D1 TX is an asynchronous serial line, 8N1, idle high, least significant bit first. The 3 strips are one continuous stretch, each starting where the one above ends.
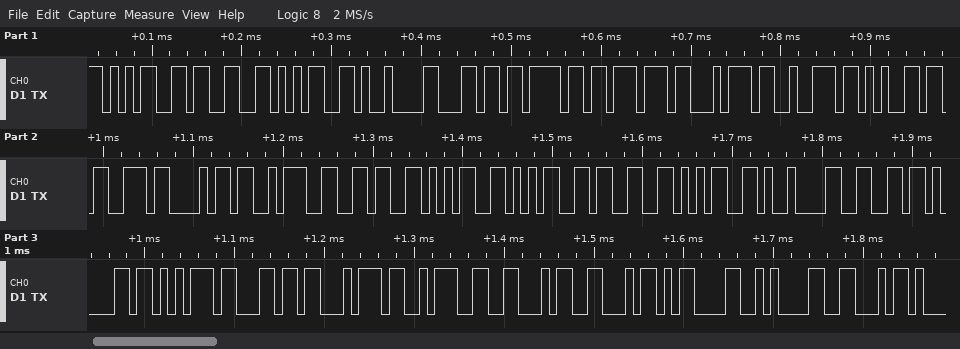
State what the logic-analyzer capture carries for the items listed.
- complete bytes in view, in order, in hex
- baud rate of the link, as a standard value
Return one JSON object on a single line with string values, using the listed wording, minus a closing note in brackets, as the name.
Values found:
{"complete bytes in view, in order, in hex": "35 33 35 09 6C 6F 77 74 72 65 73 68 3A 36 35 35 33 35 09 66 61 75 6C 74 3A 46 46 0D 0A 46", "baud rate of the link, as a standard value": "115200 baud"}
